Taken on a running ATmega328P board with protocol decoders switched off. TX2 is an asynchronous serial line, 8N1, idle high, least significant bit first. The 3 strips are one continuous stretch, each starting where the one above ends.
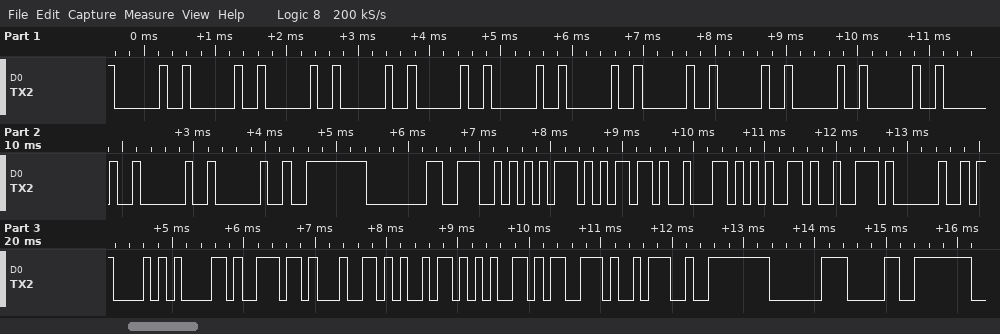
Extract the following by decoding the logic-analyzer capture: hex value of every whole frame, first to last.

20 20 20 20 20 20 20 20 20 20 20 20 20 20 FE 80 4E 75 6D 62 65 72 20 43 61 6E 64 69 65 73 3A FE C0 30
